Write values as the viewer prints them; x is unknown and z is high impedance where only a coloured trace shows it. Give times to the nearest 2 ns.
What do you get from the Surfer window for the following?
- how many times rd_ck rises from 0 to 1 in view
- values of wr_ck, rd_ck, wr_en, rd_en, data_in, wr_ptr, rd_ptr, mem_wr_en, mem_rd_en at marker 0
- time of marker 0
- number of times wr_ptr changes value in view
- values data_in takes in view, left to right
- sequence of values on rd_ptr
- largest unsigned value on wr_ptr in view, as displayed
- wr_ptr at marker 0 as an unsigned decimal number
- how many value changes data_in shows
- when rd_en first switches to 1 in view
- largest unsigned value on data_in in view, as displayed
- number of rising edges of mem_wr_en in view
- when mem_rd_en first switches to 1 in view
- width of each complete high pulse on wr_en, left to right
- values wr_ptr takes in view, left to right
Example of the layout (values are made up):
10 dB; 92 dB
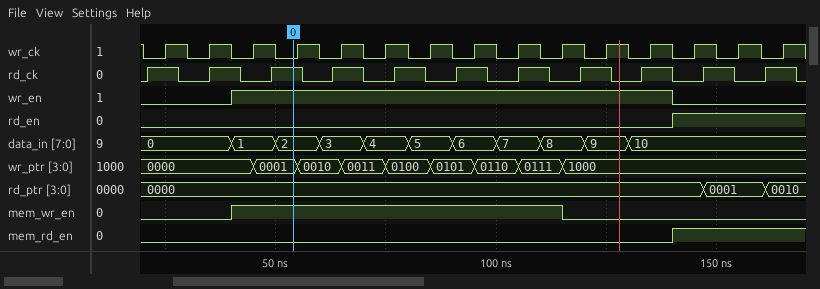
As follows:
11; wr_ck=0, rd_ck=1, wr_en=1, rd_en=0, data_in=2, wr_ptr=0001, rd_ptr=0000, mem_wr_en=1, mem_rd_en=0; 54 ns; 8; 0, 1, 2, 3, 4, 5, 6, 7, 8, 9, 10; 0000, 0001, 0010; 1000; 1; 10; 140 ns; 10; 1; 140 ns; 100 ns; 0000, 0001, 0010, 0011, 0100, 0101, 0110, 0111, 1000
